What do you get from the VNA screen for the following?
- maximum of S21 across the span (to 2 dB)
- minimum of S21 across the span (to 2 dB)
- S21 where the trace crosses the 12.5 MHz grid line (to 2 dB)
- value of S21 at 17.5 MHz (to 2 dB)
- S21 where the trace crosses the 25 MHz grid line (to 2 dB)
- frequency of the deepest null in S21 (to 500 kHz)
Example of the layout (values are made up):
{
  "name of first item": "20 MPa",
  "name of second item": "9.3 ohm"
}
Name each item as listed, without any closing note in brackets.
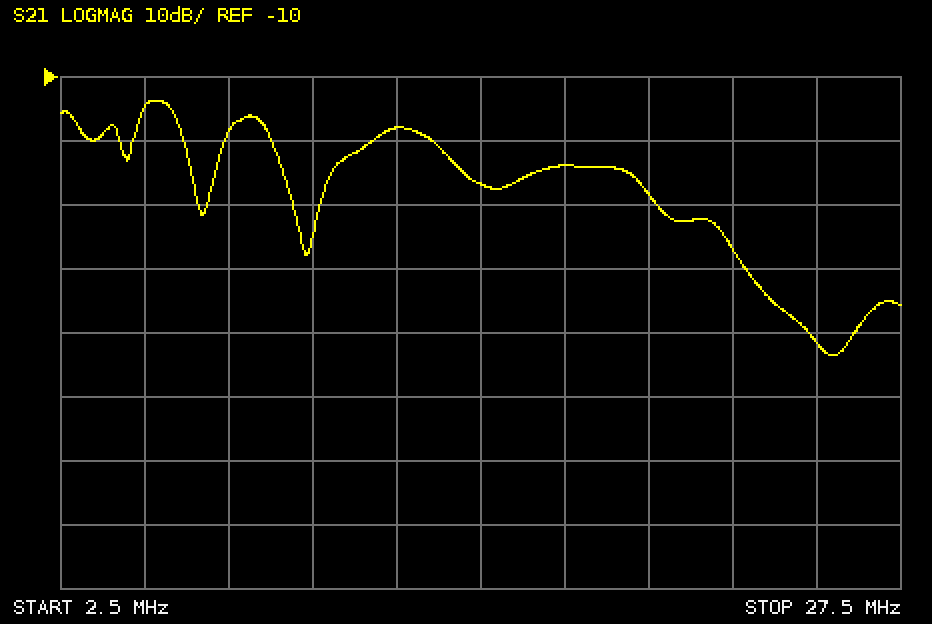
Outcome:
{
  "maximum of S21 across the span": "-14 dB",
  "minimum of S21 across the span": "-54 dB",
  "S21 where the trace crosses the 12.5 MHz grid line": "-18 dB",
  "value of S21 at 17.5 MHz": "-24 dB",
  "S21 where the trace crosses the 25 MHz grid line": "-52 dB",
  "frequency of the deepest null in S21": "25.5 MHz"
}
